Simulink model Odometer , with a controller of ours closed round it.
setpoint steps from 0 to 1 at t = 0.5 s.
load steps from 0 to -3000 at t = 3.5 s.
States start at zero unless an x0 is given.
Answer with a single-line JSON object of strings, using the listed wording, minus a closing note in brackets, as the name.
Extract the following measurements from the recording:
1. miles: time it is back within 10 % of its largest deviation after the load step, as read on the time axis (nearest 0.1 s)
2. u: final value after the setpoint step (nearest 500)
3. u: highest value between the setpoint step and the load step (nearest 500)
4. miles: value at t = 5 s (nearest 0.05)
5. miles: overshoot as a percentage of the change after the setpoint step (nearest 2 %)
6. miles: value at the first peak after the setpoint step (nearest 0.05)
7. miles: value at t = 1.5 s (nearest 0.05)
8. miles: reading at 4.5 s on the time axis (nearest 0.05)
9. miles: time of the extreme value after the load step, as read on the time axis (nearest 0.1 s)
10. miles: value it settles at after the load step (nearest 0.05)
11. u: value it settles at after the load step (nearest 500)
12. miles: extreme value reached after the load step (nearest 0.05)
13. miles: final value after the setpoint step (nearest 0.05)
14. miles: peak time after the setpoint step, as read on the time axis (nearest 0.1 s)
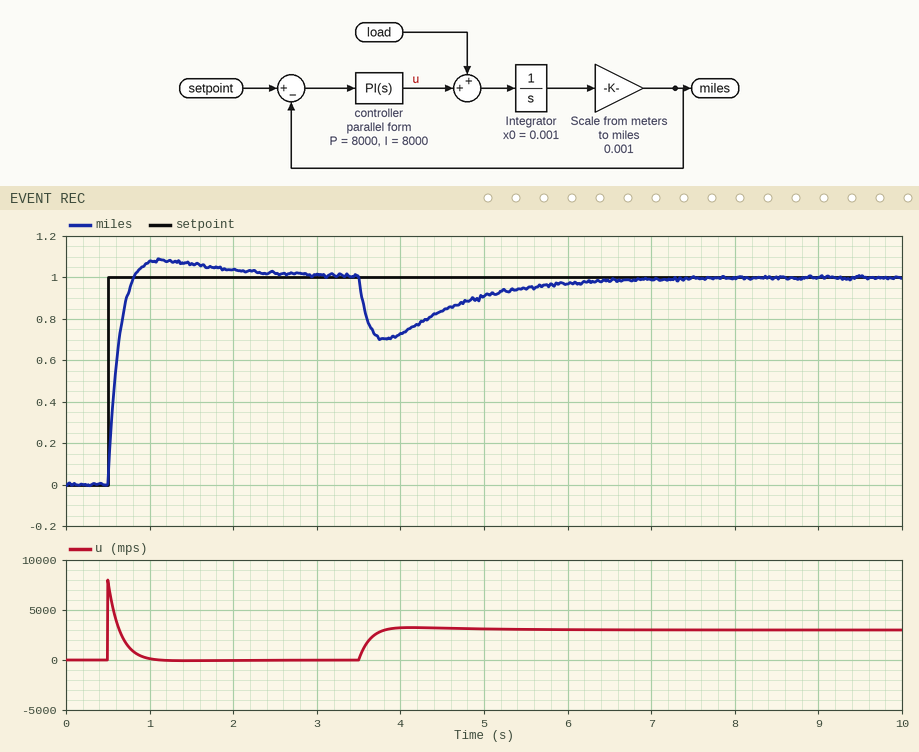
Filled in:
{"miles: time it is back within 10 % of its largest deviation after the load step, as read on the time axis": "5.9 s", "u: final value after the setpoint step": "0", "u: highest value between the setpoint step and the load step": "8000", "miles: value at t = 5 s": "0.90", "miles: overshoot as a percentage of the change after the setpoint step": "8 %", "miles: value at the first peak after the setpoint step": "1.10", "miles: value at t = 1.5 s": "1.05", "miles: reading at 4.5 s on the time axis": "0.85", "miles: time of the extreme value after the load step, as read on the time axis": "3.8 s", "miles: value it settles at after the load step": "1.00", "u: value it settles at after the load step": "3000", "miles: extreme value reached after the load step": "0.70", "miles: final value after the setpoint step": "1.00", "miles: peak time after the setpoint step, as read on the time axis": "1.1 s"}
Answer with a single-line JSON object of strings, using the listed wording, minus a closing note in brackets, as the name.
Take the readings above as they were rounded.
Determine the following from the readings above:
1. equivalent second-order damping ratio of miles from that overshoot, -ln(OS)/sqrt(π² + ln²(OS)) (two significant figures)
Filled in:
{"equivalent second-order damping ratio of miles from that overshoot, -ln(OS)/sqrt(π² + ln²(OS))": "0.63"}
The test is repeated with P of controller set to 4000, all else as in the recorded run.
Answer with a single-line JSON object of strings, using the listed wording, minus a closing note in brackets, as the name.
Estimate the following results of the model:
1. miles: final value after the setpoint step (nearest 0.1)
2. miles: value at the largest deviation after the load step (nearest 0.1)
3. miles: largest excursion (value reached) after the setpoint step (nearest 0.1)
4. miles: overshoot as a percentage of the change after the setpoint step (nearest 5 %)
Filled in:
{"miles: final value after the setpoint step": "1.0", "miles: value at the largest deviation after the load step": "0.5", "miles: largest excursion (value reached) after the setpoint step": "1.2", "miles: overshoot as a percentage of the change after the setpoint step": "20 %"}
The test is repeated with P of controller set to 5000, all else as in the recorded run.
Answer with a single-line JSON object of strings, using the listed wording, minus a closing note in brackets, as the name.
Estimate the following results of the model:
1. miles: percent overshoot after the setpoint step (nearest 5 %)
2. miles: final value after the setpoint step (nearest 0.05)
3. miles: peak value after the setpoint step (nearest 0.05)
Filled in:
{"miles: percent overshoot after the setpoint step": "15 %", "miles: final value after the setpoint step": "1.00", "miles: peak value after the setpoint step": "1.15"}
